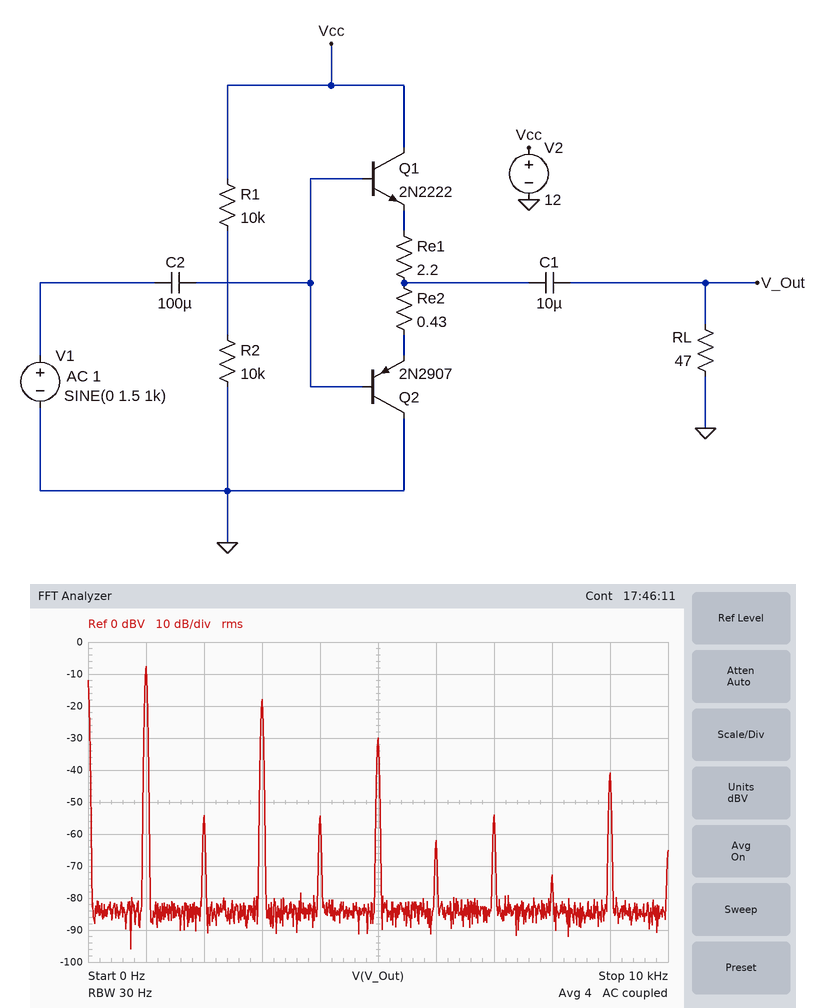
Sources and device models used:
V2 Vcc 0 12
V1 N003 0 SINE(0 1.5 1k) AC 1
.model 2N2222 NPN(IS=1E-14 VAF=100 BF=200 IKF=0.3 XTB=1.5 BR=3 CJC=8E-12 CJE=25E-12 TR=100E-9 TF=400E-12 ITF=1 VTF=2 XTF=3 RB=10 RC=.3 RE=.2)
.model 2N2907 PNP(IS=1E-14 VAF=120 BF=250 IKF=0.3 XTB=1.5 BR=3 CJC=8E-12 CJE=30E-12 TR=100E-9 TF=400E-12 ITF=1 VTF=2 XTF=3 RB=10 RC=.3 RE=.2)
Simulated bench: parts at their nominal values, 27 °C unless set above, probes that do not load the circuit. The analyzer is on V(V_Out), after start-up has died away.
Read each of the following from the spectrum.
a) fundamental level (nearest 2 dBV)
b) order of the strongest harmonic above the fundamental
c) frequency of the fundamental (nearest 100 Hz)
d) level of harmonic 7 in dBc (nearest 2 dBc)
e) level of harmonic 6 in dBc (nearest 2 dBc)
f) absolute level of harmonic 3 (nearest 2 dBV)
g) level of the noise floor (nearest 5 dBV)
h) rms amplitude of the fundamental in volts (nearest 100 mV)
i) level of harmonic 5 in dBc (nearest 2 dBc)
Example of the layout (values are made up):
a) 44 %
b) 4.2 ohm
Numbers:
a) -8 dBV
b) 3
c) 1.0 kHz
d) -46 dBc
e) -54 dBc
f) -18 dBV
g) -85 dBV
h) 400 mV
i) -22 dBc
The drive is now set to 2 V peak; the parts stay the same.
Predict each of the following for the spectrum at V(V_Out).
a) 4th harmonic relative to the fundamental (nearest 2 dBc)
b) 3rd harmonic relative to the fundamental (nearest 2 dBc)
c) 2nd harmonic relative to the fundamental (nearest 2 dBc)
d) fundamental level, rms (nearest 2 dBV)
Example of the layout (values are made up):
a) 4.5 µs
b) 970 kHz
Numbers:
a) -50 dBc
b) -14 dBc
c) -46 dBc
d) -2 dBV
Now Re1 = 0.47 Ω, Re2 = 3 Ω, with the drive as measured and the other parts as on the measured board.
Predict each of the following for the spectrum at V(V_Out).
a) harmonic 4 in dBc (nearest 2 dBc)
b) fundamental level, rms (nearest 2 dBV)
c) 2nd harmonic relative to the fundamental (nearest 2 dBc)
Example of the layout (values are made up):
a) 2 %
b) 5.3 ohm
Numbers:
a) -44 dBc
b) -8 dBV
c) -44 dBc
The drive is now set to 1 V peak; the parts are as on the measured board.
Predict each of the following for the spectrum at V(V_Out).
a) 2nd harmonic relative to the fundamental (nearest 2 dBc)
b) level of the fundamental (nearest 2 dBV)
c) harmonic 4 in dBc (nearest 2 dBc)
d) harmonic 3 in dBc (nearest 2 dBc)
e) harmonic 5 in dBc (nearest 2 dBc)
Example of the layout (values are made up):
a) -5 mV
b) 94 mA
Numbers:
a) -50 dBc
b) -18 dBV
c) -46 dBc
d) -6 dBc
e) -26 dBc
